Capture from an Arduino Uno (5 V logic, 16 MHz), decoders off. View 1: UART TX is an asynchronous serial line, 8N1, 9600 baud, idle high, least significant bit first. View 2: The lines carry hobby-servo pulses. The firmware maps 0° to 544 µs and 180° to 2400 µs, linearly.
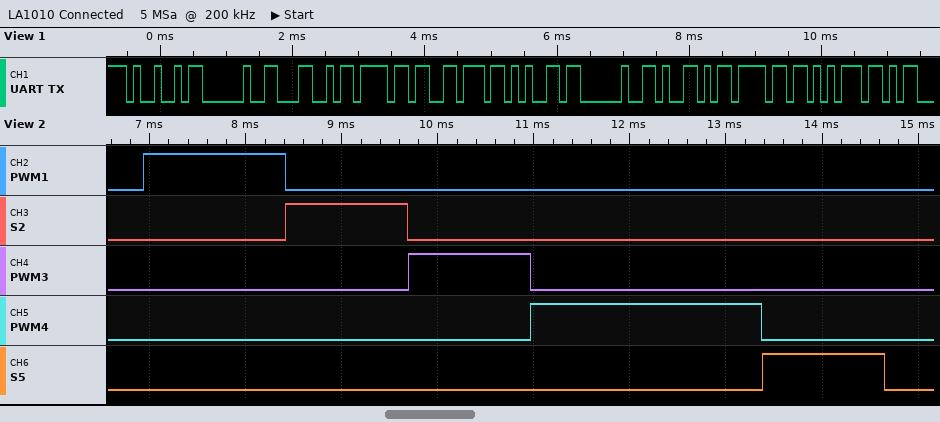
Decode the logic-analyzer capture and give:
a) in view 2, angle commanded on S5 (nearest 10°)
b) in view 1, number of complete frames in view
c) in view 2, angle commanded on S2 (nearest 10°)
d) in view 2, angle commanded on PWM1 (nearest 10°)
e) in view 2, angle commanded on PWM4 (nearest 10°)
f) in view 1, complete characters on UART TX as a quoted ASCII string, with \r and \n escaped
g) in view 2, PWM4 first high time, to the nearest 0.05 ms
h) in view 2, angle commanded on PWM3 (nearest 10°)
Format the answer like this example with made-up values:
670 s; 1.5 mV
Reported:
70°; 10; 70°; 90°; 180°; "I Love You"; 2.40 ms; 70°
